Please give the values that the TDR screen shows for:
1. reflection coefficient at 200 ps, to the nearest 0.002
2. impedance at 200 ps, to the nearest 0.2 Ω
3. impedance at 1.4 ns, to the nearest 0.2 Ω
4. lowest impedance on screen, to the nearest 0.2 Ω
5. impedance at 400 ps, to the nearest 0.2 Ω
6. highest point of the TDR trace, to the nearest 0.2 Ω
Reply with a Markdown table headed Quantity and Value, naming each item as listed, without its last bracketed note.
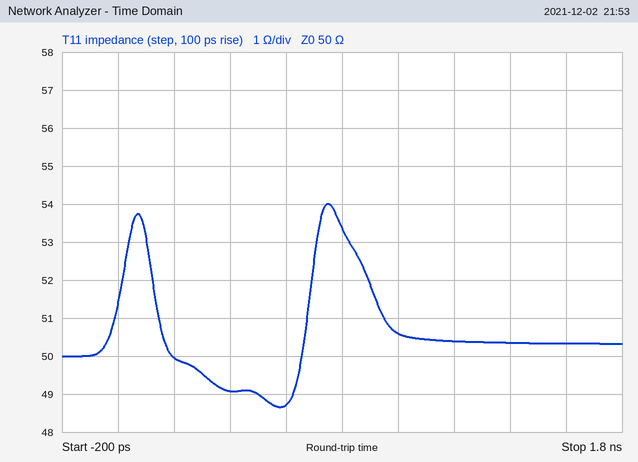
| Quantity | Value |
|---|---|
| reflection coefficient at 200 ps, to the nearest 0.002 | 0.000 |
| impedance at 200 ps, to the nearest 0.2 Ω | 50.0 Ω |
| impedance at 1.4 ns, to the nearest 0.2 Ω | 50.4 Ω |
| lowest impedance on screen, to the nearest 0.2 Ω | 48.6 Ω |
| impedance at 400 ps, to the nearest 0.2 Ω | 49.0 Ω |
| highest point of the TDR trace, to the nearest 0.2 Ω | 54.0 Ω |
